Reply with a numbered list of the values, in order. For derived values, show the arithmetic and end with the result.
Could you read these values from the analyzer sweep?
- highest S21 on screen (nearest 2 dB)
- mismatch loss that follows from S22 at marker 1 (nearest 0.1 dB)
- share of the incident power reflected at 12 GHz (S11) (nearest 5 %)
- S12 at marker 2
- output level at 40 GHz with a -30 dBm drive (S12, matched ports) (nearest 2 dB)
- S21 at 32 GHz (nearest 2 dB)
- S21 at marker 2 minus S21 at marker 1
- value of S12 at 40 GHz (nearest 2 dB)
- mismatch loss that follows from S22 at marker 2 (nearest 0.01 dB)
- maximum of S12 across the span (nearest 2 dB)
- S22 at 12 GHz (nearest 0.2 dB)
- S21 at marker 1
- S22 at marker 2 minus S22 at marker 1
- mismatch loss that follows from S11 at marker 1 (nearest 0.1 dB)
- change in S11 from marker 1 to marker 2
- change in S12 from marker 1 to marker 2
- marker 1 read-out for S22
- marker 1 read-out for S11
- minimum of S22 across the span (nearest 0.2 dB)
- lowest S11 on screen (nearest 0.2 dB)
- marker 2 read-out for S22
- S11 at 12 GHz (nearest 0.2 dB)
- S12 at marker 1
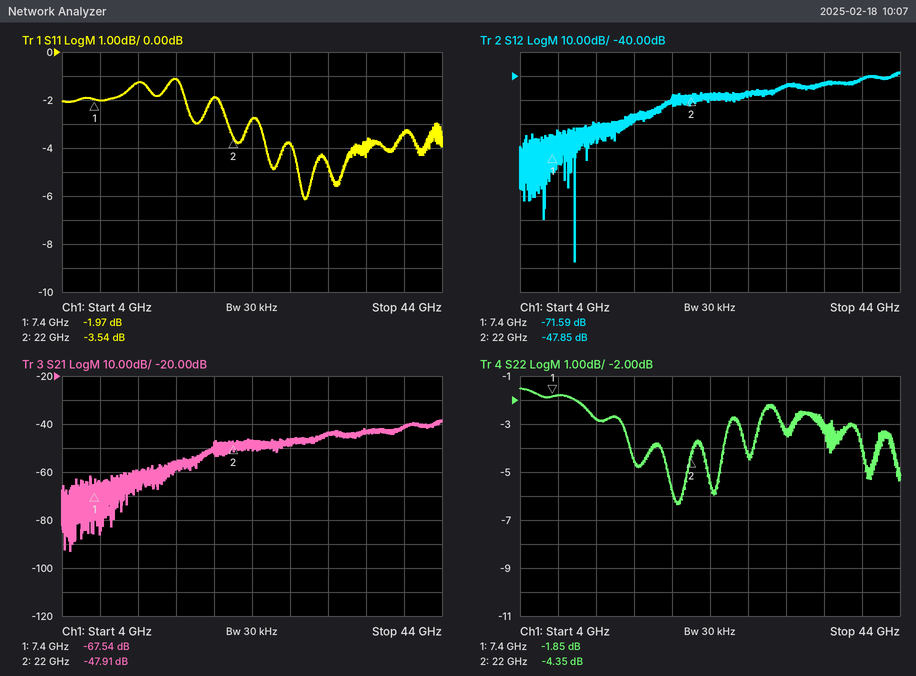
1. -38 dB
2. −10 log10(1 − 10^(-1.85/10)) ≈ 4.6 dB
3. 10^(-1.2/10) ≈ 75.9 %, so 75 % to the nearest 5 %
4. -47.85 dB
5. -30 dBm + (-42 dB) = -72 dBm
6. -44 dB
7. -47.91 − (-67.54) = 19.63 dB
8. -42 dB
9. −10 log10(1 − 10^(-4.35/10)) ≈ 1.99 dB
10. -38 dB
11. -2.8 dB
12. -67.54 dB
13. -4.35 − (-1.85) = -2.50 dB
14. −10 log10(1 − 10^(-1.97/10)) ≈ 4.4 dB
15. -3.54 − (-1.97) = -1.57 dB
16. -47.85 − (-71.59) = 23.74 dB
17. -1.85 dB
18. -1.97 dB
19. -6.4 dB
20. -6.2 dB
21. -4.35 dB
22. -1.2 dB
23. -71.59 dB
